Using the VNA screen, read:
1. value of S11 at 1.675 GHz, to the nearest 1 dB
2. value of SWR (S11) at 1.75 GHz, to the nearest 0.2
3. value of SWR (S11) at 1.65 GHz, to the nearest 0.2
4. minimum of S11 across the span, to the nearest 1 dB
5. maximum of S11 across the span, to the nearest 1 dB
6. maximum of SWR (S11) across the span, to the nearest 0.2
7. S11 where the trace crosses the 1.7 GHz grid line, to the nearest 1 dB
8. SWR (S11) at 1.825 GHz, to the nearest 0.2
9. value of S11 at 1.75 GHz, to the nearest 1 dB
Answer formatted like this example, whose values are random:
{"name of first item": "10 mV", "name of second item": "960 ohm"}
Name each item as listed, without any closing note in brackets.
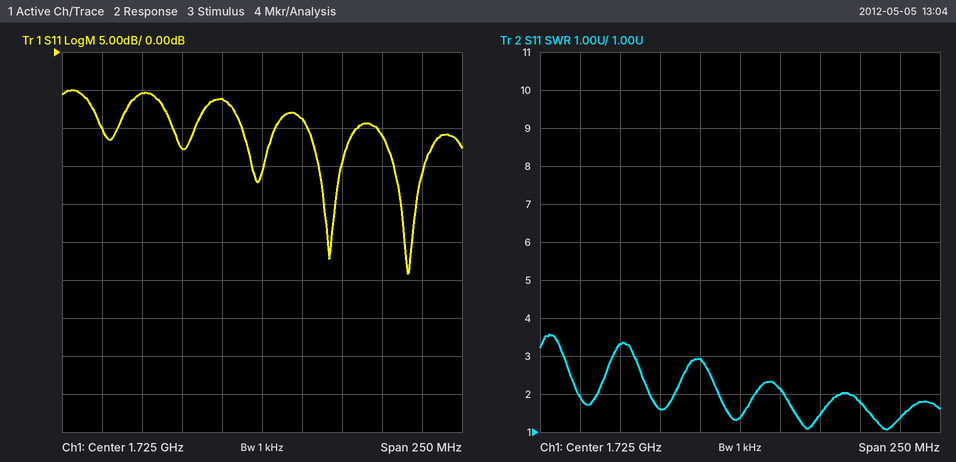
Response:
{"value of S11 at 1.675 GHz, to the nearest 1 dB": "-13 dB", "value of SWR (S11) at 1.75 GHz, to the nearest 0.2": "2.2", "value of SWR (S11) at 1.65 GHz, to the nearest 0.2": "3.4", "minimum of S11 across the span, to the nearest 1 dB": "-29 dB", "maximum of S11 across the span, to the nearest 1 dB": "-5 dB", "maximum of SWR (S11) across the span, to the nearest 0.2": "3.6", "S11 where the trace crosses the 1.7 GHz grid line, to the nearest 1 dB": "-6 dB", "SWR (S11) at 1.825 GHz, to the nearest 0.2": "1.4", "value of S11 at 1.75 GHz, to the nearest 1 dB": "-9 dB"}
